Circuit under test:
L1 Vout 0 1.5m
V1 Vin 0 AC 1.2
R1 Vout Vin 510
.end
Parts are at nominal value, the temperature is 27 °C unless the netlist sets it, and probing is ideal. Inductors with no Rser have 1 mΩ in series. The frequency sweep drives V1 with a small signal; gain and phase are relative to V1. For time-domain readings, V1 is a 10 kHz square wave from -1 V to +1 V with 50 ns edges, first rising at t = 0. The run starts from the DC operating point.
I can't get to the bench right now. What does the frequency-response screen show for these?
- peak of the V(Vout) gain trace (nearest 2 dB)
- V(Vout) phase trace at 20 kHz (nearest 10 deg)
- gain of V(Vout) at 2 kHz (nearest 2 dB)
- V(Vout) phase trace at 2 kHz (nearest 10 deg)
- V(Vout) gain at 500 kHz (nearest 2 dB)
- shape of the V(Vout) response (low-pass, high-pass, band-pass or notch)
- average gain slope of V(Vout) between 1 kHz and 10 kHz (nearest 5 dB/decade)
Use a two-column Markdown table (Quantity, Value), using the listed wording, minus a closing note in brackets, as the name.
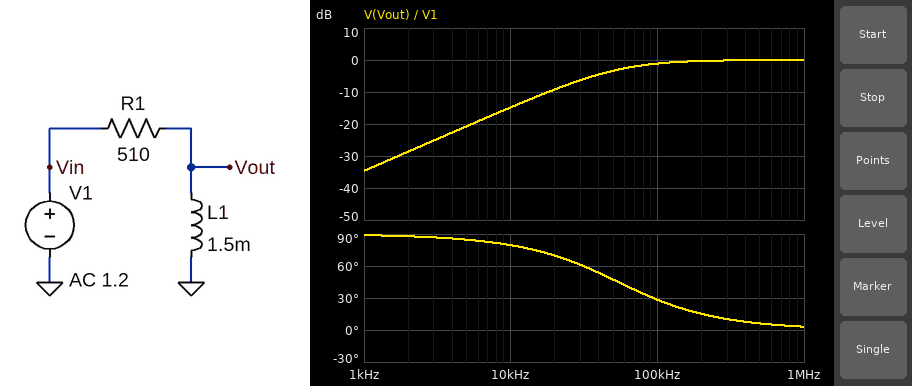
| Quantity | Value |
|---|---|
| peak of the V(Vout) gain trace | 0 dB |
| V(Vout) phase trace at 20 kHz | 70 deg |
| gain of V(Vout) at 2 kHz | -28 dB |
| V(Vout) phase trace at 2 kHz | 90 deg |
| V(Vout) gain at 500 kHz | 0 dB |
| shape of the V(Vout) response | high-pass |
| average gain slope of V(Vout) between 1 kHz and 10 kHz | 20 dB/decade |
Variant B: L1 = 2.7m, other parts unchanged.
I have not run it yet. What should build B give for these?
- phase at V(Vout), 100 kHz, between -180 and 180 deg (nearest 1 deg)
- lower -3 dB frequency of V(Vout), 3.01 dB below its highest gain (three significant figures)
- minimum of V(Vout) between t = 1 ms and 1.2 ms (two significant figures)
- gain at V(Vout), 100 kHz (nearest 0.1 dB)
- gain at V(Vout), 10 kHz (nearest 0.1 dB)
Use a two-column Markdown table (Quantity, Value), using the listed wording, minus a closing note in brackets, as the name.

| Quantity | Value |
|---|---|
| phase at V(Vout), 100 kHz, between -180 and 180 deg | 17 deg |
| lower -3 dB frequency of V(Vout), 3.01 dB below its highest gain | 30.1 kHz |
| minimum of V(Vout) between t = 1 ms and 1.2 ms | -2.0 V |
| gain at V(Vout), 100 kHz | -0.4 dB |
| gain at V(Vout), 10 kHz | -10.0 dB |
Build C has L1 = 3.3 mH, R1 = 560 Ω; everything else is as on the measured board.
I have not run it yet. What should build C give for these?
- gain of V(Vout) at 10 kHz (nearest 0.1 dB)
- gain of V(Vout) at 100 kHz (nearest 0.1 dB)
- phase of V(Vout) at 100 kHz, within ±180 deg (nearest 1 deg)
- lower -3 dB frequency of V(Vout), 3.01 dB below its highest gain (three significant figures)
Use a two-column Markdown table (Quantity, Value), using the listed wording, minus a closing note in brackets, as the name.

| Quantity | Value |
|---|---|
| gain of V(Vout) at 10 kHz | -9.2 dB |
| gain of V(Vout) at 100 kHz | -0.3 dB |
| phase of V(Vout) at 100 kHz, within ±180 deg | 15 deg |
| lower -3 dB frequency of V(Vout), 3.01 dB below its highest gain | 27.0 kHz |
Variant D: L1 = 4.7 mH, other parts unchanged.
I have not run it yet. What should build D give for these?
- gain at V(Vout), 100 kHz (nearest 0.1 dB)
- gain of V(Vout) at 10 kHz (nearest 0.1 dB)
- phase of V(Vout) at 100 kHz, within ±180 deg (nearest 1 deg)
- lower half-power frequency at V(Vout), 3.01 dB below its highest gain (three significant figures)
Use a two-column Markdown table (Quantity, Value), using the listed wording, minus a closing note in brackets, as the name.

| Quantity | Value |
|---|---|
| gain at V(Vout), 100 kHz | -0.1 dB |
| gain of V(Vout) at 10 kHz | -6.0 dB |
| phase of V(Vout) at 100 kHz, within ±180 deg | 10 deg |
| lower half-power frequency at V(Vout), 3.01 dB below its highest gain | 17.3 kHz |
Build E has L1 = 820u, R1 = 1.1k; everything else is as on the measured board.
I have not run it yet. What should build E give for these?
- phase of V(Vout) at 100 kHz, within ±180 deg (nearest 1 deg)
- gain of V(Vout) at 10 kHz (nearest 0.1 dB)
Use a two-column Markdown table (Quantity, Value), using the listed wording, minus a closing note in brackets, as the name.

| Quantity | Value |
|---|---|
| phase of V(Vout) at 100 kHz, within ±180 deg | 65 deg |
| gain of V(Vout) at 10 kHz | -26.6 dB |
